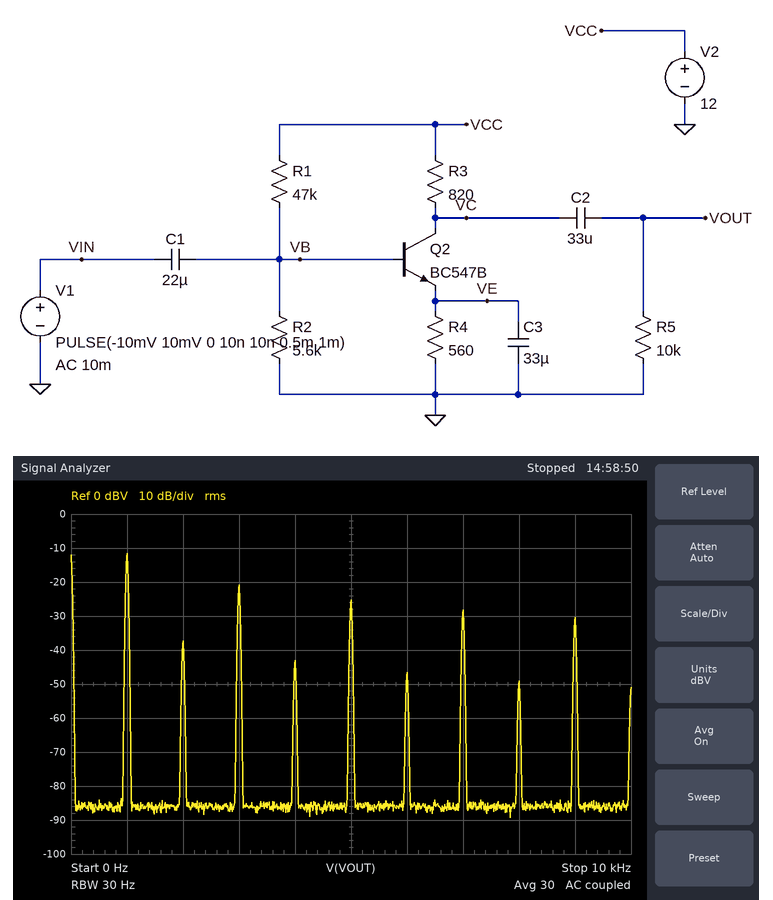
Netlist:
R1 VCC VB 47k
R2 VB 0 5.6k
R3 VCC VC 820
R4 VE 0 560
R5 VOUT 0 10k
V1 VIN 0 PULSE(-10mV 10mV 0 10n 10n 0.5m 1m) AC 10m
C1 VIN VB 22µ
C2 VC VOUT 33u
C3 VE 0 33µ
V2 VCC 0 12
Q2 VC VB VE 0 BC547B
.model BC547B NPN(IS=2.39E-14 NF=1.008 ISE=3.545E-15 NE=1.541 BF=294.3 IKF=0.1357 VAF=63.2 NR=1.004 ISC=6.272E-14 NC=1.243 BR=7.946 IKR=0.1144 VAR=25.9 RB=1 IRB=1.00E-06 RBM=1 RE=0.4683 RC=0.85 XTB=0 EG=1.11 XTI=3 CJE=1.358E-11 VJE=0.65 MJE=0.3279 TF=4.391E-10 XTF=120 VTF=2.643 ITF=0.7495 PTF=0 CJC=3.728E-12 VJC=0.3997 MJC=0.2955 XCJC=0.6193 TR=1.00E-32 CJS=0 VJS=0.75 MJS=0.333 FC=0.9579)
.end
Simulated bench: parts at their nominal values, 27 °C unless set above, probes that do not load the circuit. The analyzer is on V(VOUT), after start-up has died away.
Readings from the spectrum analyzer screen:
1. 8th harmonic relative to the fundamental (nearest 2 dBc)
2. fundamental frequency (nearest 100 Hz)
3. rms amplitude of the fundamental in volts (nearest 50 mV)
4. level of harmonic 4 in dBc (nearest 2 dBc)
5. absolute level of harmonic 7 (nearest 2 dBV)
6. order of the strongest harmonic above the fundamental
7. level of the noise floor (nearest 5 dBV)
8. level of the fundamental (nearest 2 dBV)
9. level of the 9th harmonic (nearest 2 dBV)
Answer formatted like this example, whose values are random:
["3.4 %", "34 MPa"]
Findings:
["-38 dBc", "1.0 kHz", "250 mV", "-32 dBc", "-28 dBV", "3", "-85 dBV", "-12 dBV", "-30 dBV"]
